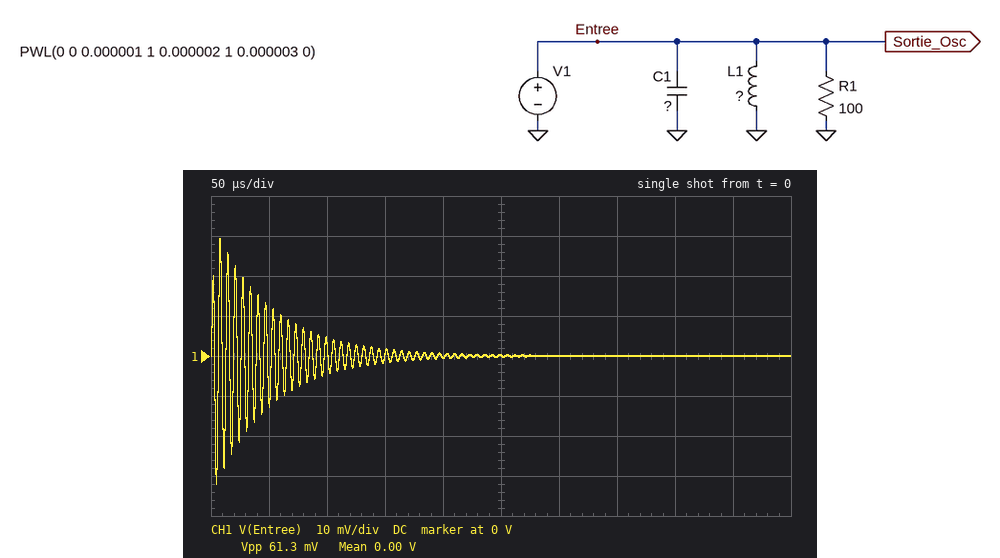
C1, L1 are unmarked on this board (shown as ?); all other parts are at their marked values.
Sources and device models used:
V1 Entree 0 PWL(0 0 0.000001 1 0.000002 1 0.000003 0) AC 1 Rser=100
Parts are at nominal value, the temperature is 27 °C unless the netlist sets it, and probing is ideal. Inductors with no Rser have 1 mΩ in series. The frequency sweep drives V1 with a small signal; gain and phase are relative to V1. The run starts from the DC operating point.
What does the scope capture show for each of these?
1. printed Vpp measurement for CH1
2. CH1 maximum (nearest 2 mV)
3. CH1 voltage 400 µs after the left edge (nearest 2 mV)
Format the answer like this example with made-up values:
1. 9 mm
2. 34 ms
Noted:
1. 61.3 mV
2. 30 mV
3. 0 V
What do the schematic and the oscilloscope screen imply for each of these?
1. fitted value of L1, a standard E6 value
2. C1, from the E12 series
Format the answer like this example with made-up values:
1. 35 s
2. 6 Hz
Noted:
1. 2.2 µH
2. 470 nF
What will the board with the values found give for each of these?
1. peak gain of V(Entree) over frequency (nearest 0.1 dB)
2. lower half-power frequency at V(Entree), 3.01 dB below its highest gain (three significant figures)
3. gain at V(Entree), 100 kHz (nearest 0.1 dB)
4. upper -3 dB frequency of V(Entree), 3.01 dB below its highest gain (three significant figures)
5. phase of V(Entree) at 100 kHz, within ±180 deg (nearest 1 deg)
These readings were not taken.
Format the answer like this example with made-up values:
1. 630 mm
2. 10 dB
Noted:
1. -6.1 dB
2. 153 kHz
3. -32.6 dB
4. 160 kHz
5. 87 deg
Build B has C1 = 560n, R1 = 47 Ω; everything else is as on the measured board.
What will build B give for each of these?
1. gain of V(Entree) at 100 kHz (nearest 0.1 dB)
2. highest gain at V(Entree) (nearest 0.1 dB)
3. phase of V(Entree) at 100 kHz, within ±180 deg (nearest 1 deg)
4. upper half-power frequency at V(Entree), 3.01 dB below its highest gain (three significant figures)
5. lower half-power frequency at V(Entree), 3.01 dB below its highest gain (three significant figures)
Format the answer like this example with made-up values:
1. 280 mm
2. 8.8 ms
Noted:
1. -31.4 dB
2. -10.0 dB
3. 85 deg
4. 148 kHz
5. 139 kHz
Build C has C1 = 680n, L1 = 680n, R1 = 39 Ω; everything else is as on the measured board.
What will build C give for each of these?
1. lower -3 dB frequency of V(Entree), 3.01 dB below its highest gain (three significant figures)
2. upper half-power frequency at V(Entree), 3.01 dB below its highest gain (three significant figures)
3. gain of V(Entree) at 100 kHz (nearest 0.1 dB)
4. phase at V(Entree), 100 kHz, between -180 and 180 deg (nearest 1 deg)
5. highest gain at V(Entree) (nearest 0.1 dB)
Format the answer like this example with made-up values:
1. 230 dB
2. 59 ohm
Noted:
1. 230 kHz
2. 238 kHz
3. -45.6 dB
4. 89 deg
5. -11.3 dB
